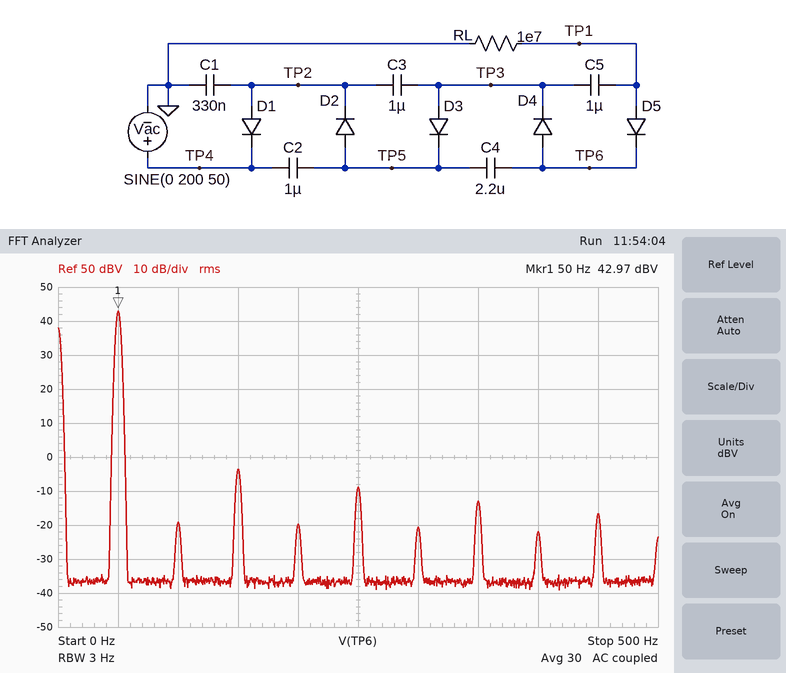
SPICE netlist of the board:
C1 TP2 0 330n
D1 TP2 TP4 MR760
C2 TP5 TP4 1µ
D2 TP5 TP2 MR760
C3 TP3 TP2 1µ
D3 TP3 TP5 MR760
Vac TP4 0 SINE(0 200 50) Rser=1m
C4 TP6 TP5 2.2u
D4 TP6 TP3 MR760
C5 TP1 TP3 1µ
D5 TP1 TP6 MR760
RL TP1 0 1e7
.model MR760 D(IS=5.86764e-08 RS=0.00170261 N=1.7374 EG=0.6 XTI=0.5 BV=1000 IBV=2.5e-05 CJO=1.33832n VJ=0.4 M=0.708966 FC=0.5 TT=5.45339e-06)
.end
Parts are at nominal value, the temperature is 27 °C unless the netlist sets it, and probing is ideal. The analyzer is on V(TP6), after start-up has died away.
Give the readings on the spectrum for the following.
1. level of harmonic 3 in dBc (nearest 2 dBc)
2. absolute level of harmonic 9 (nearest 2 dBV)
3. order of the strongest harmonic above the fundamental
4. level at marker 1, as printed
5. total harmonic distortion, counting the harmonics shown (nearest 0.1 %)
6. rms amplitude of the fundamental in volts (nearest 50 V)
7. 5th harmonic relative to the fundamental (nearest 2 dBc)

-46 dBc
-16 dBV
3
42.97 dBV
0.6 %
150 V
-52 dBc
